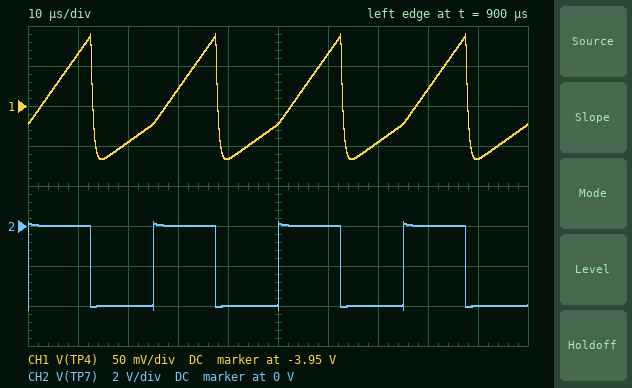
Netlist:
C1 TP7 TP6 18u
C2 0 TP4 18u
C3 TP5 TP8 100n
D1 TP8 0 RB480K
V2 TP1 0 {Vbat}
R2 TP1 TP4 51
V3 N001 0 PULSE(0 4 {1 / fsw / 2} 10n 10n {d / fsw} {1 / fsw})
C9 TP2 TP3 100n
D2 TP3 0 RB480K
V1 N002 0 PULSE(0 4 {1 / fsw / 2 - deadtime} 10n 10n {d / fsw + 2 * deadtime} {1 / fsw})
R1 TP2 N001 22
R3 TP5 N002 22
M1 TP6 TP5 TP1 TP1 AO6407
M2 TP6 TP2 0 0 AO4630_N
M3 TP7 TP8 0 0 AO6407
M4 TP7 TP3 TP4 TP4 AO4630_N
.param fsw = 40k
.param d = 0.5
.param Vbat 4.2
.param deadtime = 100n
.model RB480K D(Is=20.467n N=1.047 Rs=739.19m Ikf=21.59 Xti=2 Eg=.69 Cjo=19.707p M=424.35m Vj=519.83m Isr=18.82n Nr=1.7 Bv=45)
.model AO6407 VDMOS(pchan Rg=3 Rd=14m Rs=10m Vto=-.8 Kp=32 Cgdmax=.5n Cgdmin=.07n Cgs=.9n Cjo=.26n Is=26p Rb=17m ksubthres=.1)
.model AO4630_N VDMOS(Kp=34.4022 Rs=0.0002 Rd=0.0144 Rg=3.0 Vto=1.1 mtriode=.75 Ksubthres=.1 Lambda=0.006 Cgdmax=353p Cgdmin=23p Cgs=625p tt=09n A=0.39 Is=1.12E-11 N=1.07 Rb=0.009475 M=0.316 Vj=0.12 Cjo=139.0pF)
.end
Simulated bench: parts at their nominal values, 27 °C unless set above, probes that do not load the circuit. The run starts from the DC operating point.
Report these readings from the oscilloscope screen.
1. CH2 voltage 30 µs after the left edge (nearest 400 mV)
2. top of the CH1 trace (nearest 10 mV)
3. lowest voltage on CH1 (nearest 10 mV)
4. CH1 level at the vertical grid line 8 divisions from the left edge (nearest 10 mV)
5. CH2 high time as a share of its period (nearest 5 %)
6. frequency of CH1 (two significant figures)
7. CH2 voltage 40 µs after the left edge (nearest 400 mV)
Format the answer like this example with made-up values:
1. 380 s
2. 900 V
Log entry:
1. 0 V
2. -3.86 V
3. -4.02 V
4. -3.93 V
5. 50 %
6. 40 kHz
7. -4.0 V
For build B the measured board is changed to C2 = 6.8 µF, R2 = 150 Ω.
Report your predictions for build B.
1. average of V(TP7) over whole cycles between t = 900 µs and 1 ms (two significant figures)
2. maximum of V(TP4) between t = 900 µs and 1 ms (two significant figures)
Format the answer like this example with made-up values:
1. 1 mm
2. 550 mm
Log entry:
1. -2.1 V
2. -4.0 V
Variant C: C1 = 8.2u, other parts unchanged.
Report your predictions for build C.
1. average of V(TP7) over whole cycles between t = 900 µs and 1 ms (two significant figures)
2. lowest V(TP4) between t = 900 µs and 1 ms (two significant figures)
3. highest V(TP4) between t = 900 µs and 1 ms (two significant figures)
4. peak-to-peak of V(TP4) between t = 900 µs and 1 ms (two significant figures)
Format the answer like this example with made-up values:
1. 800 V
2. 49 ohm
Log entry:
1. -1.9 V
2. -3.8 V
3. -3.6 V
4. 170 mV
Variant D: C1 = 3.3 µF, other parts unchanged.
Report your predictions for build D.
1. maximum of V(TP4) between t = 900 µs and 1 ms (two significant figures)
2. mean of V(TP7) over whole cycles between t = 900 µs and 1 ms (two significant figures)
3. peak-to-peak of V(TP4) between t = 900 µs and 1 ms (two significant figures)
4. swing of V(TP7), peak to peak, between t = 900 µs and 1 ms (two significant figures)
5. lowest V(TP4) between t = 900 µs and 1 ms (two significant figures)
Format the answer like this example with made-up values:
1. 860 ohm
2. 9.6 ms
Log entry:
1. -3.0 V
2. -1.6 V
3. 180 mV
4. 4.2 V
5. -3.2 V
